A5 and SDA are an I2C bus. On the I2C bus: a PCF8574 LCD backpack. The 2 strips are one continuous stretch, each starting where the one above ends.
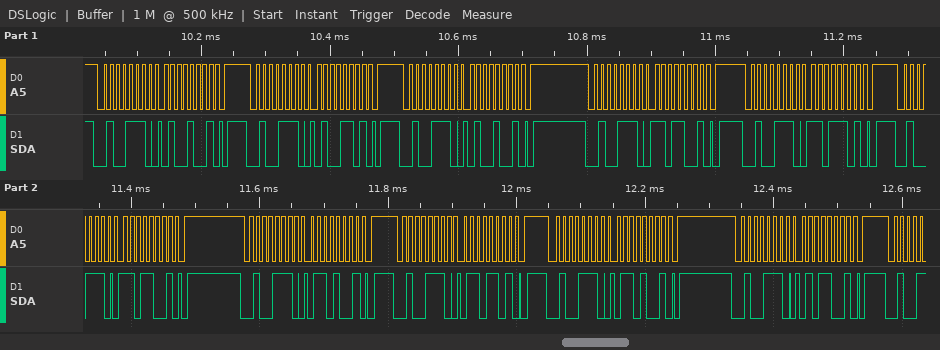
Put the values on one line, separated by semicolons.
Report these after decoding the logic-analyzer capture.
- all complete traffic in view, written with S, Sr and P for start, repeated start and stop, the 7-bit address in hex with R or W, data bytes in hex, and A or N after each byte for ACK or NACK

S 27W A 49 A P S 27W A 4D A P S 27W A 49 A P S 27W A D9 A P S 27W A DD A P S 27W A D9 A P S 27W A 69 A P S 27W A 6D A P S 27W A 69 A P S 27W A 59 A P
